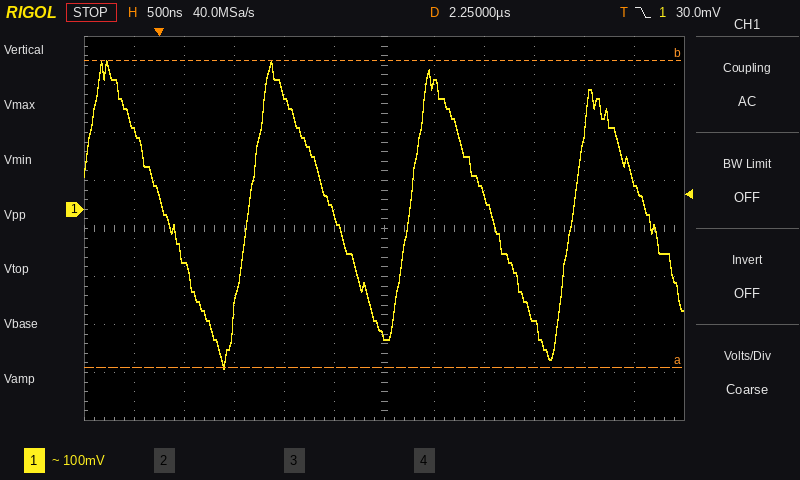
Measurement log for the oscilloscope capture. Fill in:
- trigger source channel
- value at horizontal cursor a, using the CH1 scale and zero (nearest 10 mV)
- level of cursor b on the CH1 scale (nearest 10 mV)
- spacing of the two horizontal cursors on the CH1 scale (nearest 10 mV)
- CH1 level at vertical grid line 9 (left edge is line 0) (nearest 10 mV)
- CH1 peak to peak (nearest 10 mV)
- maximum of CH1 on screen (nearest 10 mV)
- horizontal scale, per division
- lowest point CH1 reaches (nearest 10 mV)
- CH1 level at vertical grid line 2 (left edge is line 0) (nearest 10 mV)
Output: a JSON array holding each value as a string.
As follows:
["CH1", "-330 mV", "310 mV", "640 mV", "-230 mV", "640 mV", "310 mV", "500 ns", "-330 mV", "-110 mV"]
